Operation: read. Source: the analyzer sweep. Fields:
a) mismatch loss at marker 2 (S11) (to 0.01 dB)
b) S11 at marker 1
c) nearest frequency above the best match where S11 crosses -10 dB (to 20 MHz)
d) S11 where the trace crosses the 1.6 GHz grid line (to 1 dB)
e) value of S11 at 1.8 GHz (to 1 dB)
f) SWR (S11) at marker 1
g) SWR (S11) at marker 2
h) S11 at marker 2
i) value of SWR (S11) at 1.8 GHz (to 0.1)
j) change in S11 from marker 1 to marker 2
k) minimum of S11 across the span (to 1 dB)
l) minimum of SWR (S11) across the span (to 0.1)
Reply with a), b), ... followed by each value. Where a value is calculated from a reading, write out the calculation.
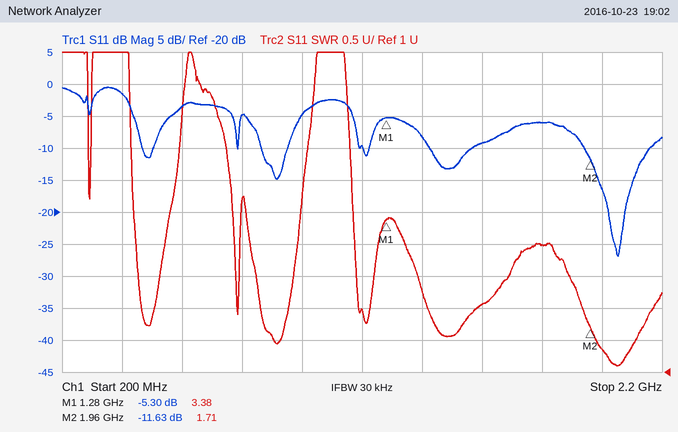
a) −10 log10(1 − 10^(-11.63/10)) ≈ 0.31 dB
b) -5.30 dB
c) 2.16 GHz
d) -9 dB
e) -6 dB
f) 3.38
g) 1.71
h) -11.63 dB
i) 3.0
j) -11.63 − (-5.3) = -6.33 dB
k) -27 dB
l) 1.1
